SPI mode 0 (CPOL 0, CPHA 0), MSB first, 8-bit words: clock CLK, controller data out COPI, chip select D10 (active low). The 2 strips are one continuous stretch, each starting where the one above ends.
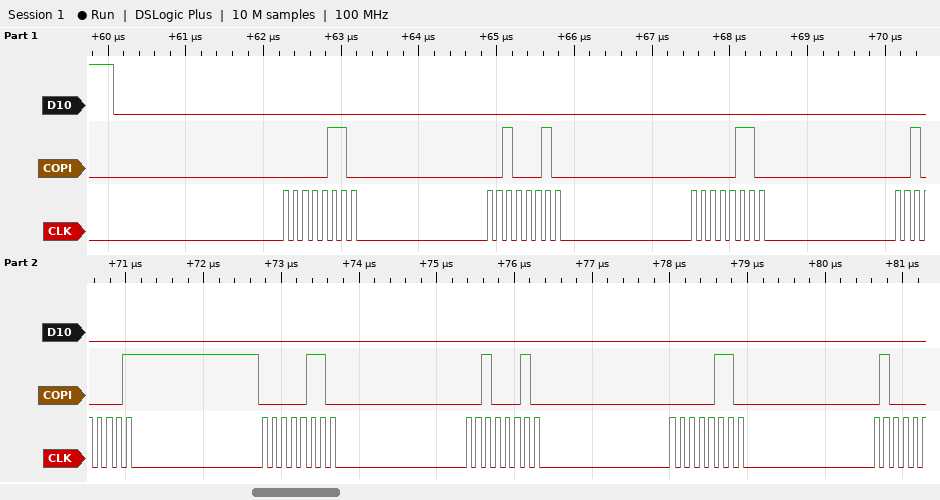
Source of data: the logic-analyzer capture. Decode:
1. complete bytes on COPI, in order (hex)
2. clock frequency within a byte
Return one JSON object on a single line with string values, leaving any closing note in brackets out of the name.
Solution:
{"complete bytes on COPI, in order": "0x06 0x22 0x06 0x21 0x06 0x22 0x06", "clock frequency within a byte": "8 MHz"}
